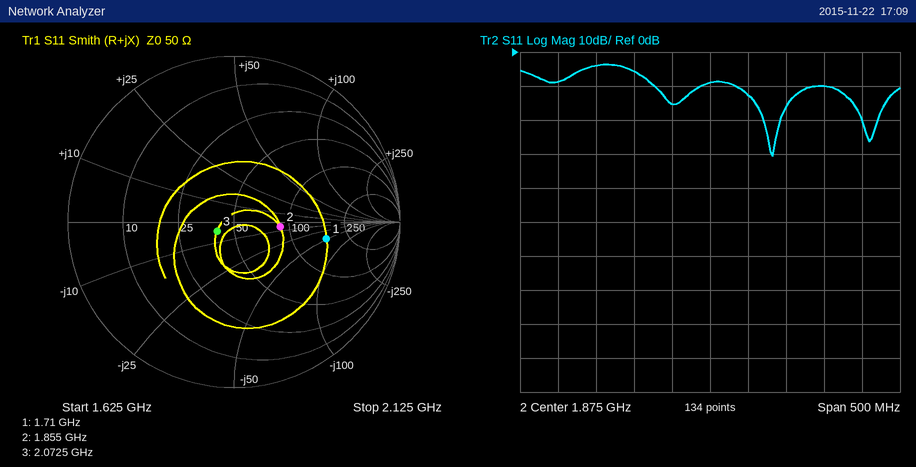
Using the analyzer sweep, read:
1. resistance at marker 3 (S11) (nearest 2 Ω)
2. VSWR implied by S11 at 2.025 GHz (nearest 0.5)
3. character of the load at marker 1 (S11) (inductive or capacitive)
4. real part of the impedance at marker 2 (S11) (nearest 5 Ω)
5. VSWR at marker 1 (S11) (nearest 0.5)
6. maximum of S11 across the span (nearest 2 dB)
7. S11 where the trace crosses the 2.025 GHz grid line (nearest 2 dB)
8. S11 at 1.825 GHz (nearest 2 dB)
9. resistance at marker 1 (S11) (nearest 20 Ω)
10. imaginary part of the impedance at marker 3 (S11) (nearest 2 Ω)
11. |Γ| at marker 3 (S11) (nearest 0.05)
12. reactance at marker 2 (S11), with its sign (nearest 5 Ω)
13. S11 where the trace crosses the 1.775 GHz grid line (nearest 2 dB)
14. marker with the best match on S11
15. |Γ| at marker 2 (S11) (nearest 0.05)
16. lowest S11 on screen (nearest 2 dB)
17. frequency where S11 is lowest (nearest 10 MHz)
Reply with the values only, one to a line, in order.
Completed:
40 Ω
2.0
capacitive
90 Ω
3.5
-4 dB
-10 dB
-16 dB
160 Ω
-4 Ω
0.10
-5 Ω
-6 dB
marker 3
0.30
-30 dB
1.96 GHz
